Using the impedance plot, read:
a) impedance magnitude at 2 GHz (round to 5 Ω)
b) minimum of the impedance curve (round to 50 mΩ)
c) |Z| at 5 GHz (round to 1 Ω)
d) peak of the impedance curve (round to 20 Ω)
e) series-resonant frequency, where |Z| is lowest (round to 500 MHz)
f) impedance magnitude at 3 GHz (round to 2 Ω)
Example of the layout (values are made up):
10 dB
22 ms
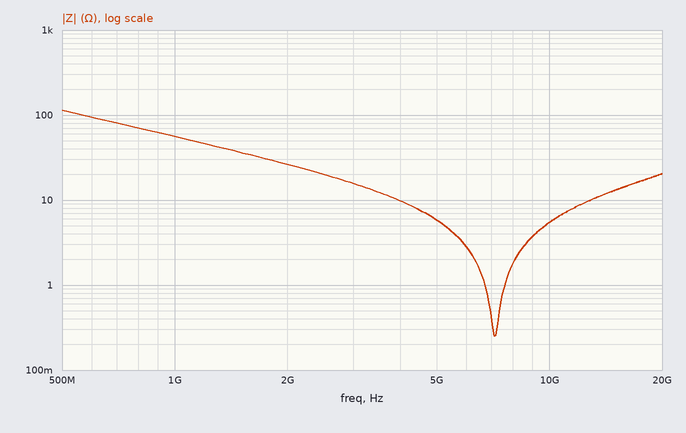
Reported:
25 Ω
250 mΩ
6 Ω
120 Ω
7.0 GHz
16 Ω
